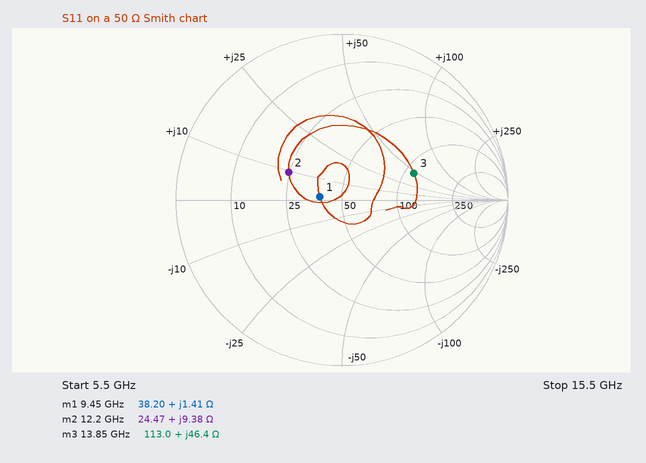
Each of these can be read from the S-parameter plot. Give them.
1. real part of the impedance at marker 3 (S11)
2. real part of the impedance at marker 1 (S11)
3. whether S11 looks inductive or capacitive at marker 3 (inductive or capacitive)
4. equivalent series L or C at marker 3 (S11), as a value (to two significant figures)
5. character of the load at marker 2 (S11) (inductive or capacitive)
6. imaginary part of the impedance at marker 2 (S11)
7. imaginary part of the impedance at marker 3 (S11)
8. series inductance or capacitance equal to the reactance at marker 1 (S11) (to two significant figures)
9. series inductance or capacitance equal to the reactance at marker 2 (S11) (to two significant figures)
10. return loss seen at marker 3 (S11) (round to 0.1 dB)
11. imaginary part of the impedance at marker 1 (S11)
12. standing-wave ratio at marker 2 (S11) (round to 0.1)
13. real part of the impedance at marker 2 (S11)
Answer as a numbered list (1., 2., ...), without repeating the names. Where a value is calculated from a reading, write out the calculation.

1. 113.0 Ω
2. 38.20 Ω
3. inductive
4. L = 46.4 Ω/(2π × 13.85 GHz) ≈ 533 pH, so 530 pH to two significant figures
5. inductive
6. +9.38 Ω
7. +46.4 Ω
8. L = 1.41 Ω/(2π × 9.45 GHz) ≈ 24 pH
9. L = 9.38 Ω/(2π × 12.2 GHz) ≈ 122 pH, so 120 pH to two significant figures
10. 6.7 dB
11. +1.41 Ω
12. 2.1
13. 24.47 Ω
